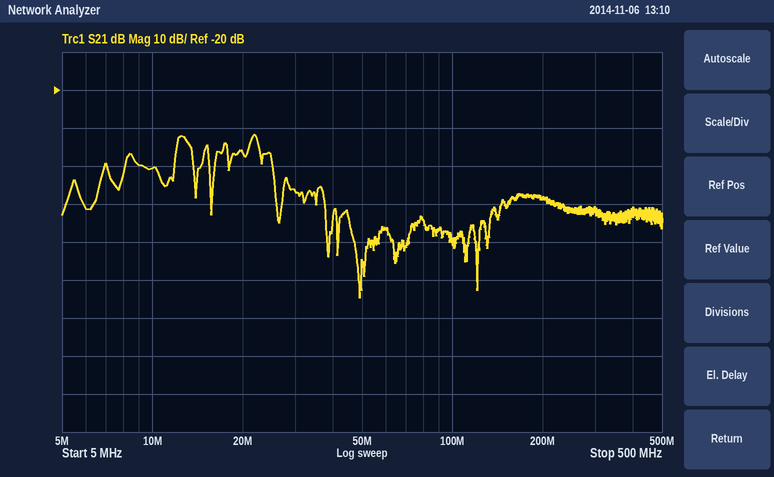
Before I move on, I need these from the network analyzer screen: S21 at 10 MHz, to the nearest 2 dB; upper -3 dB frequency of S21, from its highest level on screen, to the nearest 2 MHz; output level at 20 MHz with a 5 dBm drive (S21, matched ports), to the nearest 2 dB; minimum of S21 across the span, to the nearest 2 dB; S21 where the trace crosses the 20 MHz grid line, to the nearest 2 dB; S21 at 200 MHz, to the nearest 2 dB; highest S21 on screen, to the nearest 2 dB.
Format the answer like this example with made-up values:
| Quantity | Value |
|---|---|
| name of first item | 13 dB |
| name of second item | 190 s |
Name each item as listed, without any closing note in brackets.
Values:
| Quantity | Value |
|---|---|
| S21 at 10 MHz, to the nearest 2 dB | -40 dB |
| upper -3 dB frequency of S21, from its highest level on screen, to the nearest 2 MHz | 22 MHz |
| output level at 20 MHz with a 5 dBm drive (S21, matched ports), to the nearest 2 dB | -32 dBm |
| minimum of S21 across the span, to the nearest 2 dB | -74 dB |
| S21 where the trace crosses the 20 MHz grid line, to the nearest 2 dB | -36 dB |
| S21 at 200 MHz, to the nearest 2 dB | -48 dB |
| highest S21 on screen, to the nearest 2 dB | -32 dB |
